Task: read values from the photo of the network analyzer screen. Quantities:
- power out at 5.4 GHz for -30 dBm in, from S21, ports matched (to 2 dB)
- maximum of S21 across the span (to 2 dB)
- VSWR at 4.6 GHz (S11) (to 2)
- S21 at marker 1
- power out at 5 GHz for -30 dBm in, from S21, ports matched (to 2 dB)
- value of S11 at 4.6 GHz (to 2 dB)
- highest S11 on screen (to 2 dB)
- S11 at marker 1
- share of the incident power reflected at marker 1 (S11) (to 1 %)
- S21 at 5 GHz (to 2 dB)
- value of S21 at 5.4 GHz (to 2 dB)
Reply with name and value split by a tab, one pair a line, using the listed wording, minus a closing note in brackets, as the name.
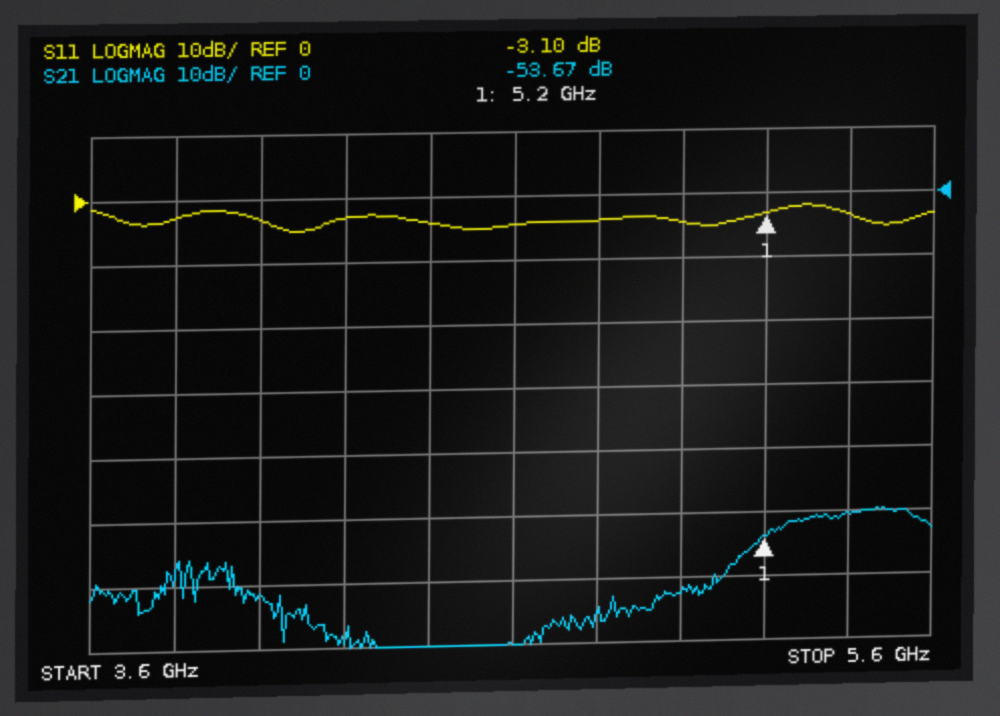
power out at 5.4 GHz for -30 dBm in, from S21, ports matched	-80 dBm
maximum of S21 across the span	-50 dB
VSWR at 4.6 GHz (S11)	4
S21 at marker 1	-53.67 dB
power out at 5 GHz for -30 dBm in, from S21, ports matched	-92 dBm
value of S11 at 4.6 GHz	-4 dB
highest S11 on screen	-2 dB
S11 at marker 1	-3.10 dB
share of the incident power reflected at marker 1 (S11)	49 %
S21 at 5 GHz	-62 dB
value of S21 at 5.4 GHz	-50 dB
